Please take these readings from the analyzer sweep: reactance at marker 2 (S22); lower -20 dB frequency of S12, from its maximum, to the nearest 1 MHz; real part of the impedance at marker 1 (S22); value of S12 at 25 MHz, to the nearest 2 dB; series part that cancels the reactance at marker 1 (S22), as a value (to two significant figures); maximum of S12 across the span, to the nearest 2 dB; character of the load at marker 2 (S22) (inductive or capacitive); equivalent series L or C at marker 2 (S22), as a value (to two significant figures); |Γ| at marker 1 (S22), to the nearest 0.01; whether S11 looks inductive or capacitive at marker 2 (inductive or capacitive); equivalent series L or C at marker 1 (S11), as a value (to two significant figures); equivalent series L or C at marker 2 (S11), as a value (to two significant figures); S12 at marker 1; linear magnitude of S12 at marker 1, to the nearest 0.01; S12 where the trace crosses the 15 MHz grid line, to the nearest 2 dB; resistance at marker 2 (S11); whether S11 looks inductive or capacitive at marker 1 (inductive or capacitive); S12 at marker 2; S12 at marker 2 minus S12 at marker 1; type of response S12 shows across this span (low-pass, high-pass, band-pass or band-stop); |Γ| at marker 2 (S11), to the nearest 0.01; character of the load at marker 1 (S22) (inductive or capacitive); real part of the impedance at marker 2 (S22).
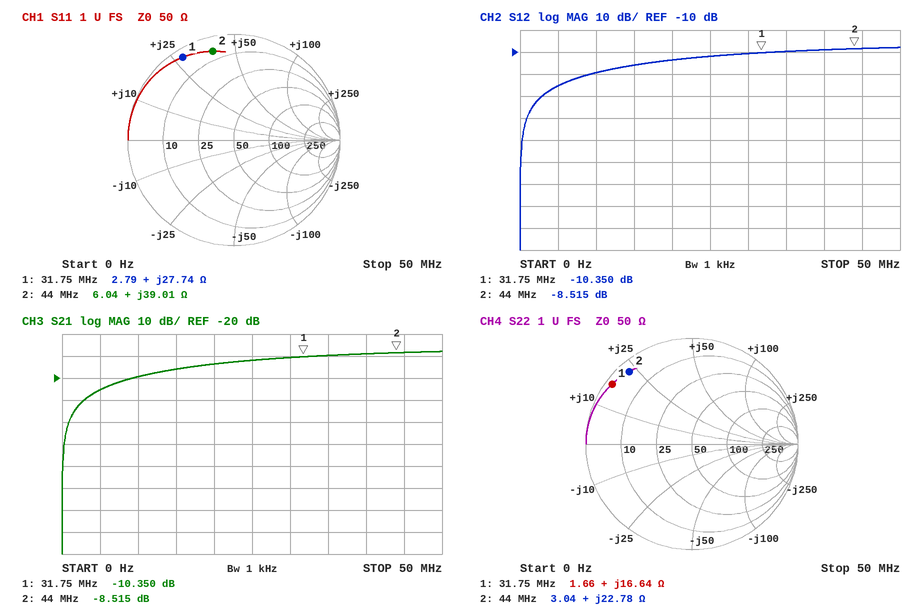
+22.78 Ω
4 MHz
1.66 Ω
-12 dB
300 pF
-8 dB
inductive
82 nH
0.94
inductive
140 nH
140 nH
-10.350 dB
0.30
-16 dB
6.04 Ω
inductive
-8.515 dB
1.835 dB
high-pass
0.86
inductive
3.04 Ω
